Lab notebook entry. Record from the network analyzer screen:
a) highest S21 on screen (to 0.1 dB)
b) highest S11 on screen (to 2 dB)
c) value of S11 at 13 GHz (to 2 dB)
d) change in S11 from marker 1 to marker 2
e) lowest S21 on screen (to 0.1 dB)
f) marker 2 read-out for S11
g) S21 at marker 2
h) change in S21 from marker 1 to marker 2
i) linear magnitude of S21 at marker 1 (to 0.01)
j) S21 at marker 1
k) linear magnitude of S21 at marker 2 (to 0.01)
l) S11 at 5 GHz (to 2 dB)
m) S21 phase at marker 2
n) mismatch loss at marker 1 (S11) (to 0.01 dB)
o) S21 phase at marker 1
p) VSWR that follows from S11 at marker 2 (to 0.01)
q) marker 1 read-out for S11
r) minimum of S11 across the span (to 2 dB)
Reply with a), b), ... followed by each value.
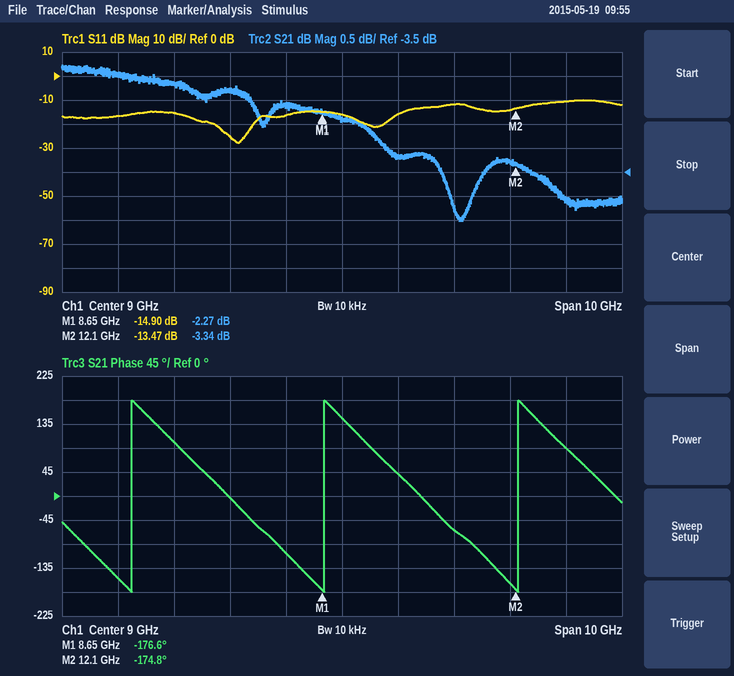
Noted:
a) -1.3 dB
b) -10 dB
c) -10 dB
d) 1.43 dB
e) -4.5 dB
f) -13.47 dB
g) -3.34 dB
h) -1.07 dB
i) 0.77
j) -2.27 dB
k) 0.68
l) -16 dB
m) -174.8°
n) 0.14 dB
o) -176.6°
p) 1.54
q) -14.90 dB
r) -28 dB
